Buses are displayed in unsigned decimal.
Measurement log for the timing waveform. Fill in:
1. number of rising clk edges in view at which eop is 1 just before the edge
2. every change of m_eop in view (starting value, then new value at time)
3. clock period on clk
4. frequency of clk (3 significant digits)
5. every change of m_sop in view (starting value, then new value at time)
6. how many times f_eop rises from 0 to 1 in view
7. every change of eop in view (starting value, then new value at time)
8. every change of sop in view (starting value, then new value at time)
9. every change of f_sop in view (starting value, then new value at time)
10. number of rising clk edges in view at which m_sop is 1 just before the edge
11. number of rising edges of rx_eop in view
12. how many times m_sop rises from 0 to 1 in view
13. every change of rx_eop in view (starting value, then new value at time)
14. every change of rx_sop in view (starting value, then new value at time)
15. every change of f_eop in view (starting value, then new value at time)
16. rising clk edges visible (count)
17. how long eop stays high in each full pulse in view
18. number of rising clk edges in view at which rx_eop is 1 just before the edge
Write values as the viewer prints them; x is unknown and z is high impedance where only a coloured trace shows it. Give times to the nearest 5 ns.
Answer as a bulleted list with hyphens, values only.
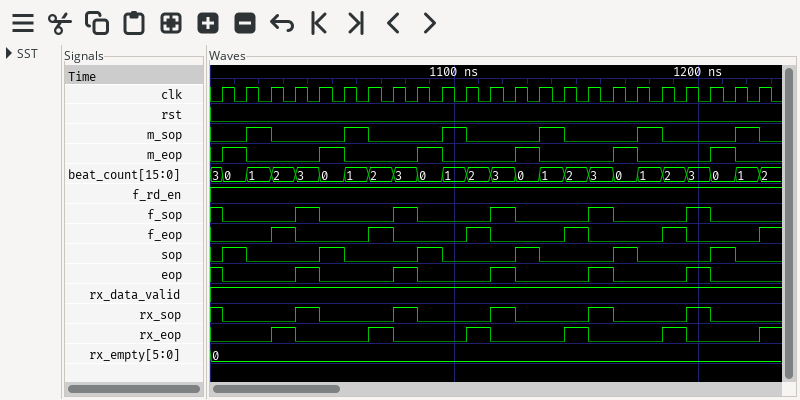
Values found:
- 6
- 0, 1 at 1005 ns, 0 at 1015 ns, 1 at 1045 ns, 0 at 1055 ns, 1 at 1085 ns, 0 at 1095 ns, 1 at 1125 ns, 0 at 1135 ns, 1 at 1165 ns, 0 at 1175 ns, 1 at 1205 ns, 0 at 1215 ns
- 10 ns
- 100 MHz
- 0, 1 at 1015 ns, 0 at 1025 ns, 1 at 1055 ns, 0 at 1065 ns, 1 at 1095 ns, 0 at 1105 ns, 1 at 1135 ns, 0 at 1145 ns, 1 at 1175 ns, 0 at 1185 ns, 1 at 1215 ns, 0 at 1225 ns
- 6
- 1, 0 at 1005 ns, 1 at 1035 ns, 0 at 1045 ns, 1 at 1075 ns, 0 at 1085 ns, 1 at 1115 ns, 0 at 1125 ns, 1 at 1155 ns, 0 at 1165 ns, 1 at 1195 ns, 0 at 1205 ns
- 0, 1 at 1005 ns, 0 at 1015 ns, 1 at 1045 ns, 0 at 1055 ns, 1 at 1085 ns, 0 at 1095 ns, 1 at 1125 ns, 0 at 1135 ns, 1 at 1165 ns, 0 at 1175 ns, 1 at 1205 ns, 0 at 1215 ns
- 1, 0 at 1005 ns, 1 at 1035 ns, 0 at 1045 ns, 1 at 1075 ns, 0 at 1085 ns, 1 at 1115 ns, 0 at 1125 ns, 1 at 1155 ns, 0 at 1165 ns, 1 at 1195 ns, 0 at 1205 ns
- 6
- 6
- 6
- 0, 1 at 1025 ns, 0 at 1035 ns, 1 at 1065 ns, 0 at 1075 ns, 1 at 1105 ns, 0 at 1115 ns, 1 at 1145 ns, 0 at 1155 ns, 1 at 1185 ns, 0 at 1195 ns, 1 at 1225 ns
- 1, 0 at 1005 ns, 1 at 1035 ns, 0 at 1045 ns, 1 at 1075 ns, 0 at 1085 ns, 1 at 1115 ns, 0 at 1125 ns, 1 at 1155 ns, 0 at 1165 ns, 1 at 1195 ns, 0 at 1205 ns
- 0, 1 at 1025 ns, 0 at 1035 ns, 1 at 1065 ns, 0 at 1075 ns, 1 at 1105 ns, 0 at 1115 ns, 1 at 1145 ns, 0 at 1155 ns, 1 at 1185 ns, 0 at 1195 ns, 1 at 1225 ns
- 23
- 10 ns, 10 ns, 10 ns, 10 ns, 10 ns
- 5
